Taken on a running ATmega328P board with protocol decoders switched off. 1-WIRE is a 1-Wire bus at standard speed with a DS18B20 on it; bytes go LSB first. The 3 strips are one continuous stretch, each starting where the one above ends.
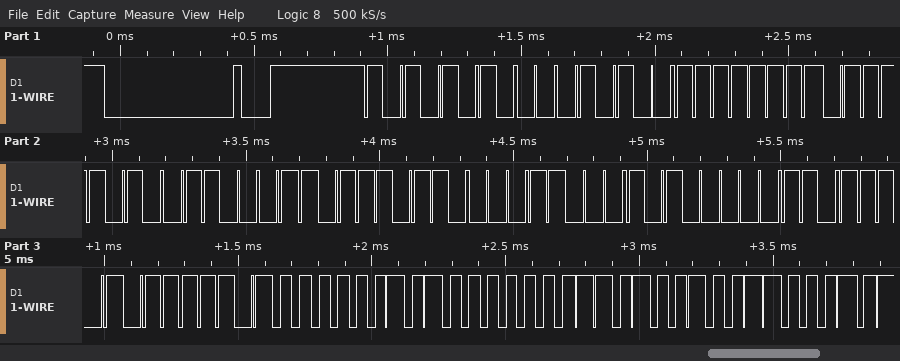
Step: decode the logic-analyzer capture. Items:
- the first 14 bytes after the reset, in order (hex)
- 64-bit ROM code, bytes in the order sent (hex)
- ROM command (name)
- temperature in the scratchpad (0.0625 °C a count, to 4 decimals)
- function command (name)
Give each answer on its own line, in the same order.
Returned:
55 28 FF 5E C6 6E 18 05 BB BE 40 01 4B 46
28 FF 5E C6 6E 18 05 BB
Match ROM
20.0000 °C
Read Scratchpad
